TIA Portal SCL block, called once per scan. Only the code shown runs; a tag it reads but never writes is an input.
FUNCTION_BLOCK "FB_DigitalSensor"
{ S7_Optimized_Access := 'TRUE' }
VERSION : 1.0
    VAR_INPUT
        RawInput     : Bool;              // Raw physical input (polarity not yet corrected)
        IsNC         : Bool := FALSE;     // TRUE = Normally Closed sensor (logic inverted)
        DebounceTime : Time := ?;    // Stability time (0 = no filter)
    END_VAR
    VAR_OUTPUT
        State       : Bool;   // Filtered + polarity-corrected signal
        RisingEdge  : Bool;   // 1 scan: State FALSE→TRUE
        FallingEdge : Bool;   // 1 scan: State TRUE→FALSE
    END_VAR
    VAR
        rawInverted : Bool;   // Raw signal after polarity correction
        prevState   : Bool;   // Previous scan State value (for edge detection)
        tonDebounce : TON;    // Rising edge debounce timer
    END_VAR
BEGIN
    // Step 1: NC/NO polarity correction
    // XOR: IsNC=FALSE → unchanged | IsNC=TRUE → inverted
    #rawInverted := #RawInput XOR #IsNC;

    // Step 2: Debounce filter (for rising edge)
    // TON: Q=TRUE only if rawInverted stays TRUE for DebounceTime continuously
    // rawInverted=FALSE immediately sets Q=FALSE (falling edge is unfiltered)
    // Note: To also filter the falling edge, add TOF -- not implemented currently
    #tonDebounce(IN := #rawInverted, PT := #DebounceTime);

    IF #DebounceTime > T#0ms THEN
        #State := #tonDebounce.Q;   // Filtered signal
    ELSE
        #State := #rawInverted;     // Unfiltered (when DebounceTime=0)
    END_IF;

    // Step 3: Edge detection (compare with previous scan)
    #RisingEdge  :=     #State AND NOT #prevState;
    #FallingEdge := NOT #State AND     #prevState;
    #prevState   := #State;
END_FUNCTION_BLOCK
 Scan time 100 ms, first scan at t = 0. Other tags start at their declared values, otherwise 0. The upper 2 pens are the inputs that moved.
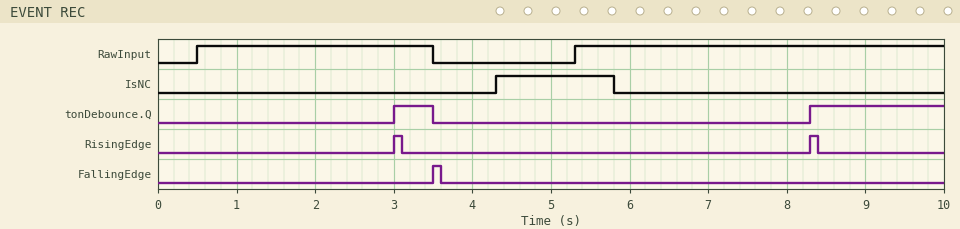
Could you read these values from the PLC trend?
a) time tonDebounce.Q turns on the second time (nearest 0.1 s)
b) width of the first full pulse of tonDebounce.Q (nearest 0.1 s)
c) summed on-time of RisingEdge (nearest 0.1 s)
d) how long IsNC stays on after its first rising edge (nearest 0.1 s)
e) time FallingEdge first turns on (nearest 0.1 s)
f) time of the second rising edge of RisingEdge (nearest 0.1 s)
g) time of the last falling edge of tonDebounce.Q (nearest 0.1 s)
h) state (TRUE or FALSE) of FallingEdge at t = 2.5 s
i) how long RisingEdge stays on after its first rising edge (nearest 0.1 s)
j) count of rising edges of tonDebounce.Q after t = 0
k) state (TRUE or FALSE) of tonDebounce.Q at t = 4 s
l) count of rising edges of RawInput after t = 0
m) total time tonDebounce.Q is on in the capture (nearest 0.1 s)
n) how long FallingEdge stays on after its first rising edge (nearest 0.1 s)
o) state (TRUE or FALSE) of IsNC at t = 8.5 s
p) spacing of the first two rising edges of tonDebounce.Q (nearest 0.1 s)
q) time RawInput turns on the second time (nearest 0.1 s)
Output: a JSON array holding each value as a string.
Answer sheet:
["8.3 s", "0.5 s", "0.2 s", "1.5 s", "3.5 s", "8.3 s", "3.5 s", "FALSE", "0.1 s", "2", "FALSE", "2", "2.2 s", "0.1 s", "FALSE", "5.3 s", "5.3 s"]
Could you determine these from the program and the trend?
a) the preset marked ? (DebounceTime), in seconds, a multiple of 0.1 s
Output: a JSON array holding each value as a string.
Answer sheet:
["2.5 s"]
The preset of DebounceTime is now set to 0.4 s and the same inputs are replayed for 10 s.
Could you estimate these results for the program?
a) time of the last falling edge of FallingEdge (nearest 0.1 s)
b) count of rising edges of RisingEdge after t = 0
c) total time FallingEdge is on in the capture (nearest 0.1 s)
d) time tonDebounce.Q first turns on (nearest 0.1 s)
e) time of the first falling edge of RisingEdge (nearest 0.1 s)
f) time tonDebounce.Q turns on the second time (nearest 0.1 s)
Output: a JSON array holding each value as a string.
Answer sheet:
["5.4 s", "3", "0.2 s", "0.9 s", "1.0 s", "4.7 s"]
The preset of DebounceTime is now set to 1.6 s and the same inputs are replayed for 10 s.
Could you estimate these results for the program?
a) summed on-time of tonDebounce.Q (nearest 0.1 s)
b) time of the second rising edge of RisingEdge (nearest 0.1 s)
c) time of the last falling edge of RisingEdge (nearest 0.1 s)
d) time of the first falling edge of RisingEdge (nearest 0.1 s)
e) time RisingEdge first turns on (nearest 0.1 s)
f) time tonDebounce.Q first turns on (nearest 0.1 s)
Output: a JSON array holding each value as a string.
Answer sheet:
["4.0 s", "7.4 s", "7.5 s", "2.2 s", "2.1 s", "2.1 s"]
